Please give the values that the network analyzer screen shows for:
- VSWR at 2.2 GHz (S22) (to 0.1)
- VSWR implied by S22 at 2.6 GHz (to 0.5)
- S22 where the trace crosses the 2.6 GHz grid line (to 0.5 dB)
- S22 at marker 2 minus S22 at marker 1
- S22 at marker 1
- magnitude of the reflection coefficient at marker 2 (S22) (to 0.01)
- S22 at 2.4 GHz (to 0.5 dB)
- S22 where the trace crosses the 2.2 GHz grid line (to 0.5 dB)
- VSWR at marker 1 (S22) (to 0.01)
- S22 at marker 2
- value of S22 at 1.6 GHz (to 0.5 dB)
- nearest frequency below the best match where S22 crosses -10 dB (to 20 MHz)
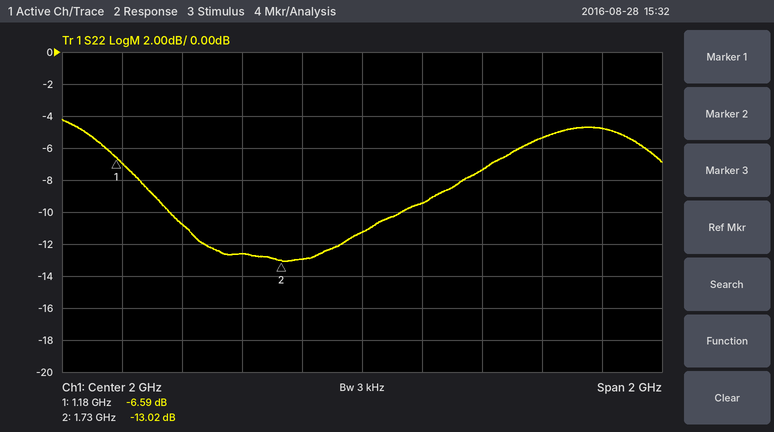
2.0
3.5
-5.5 dB
-6.43 dB
-6.59 dB
0.22
-7.5 dB
-9.5 dB
2.76
-13.02 dB
-12.5 dB
1.36 GHz
